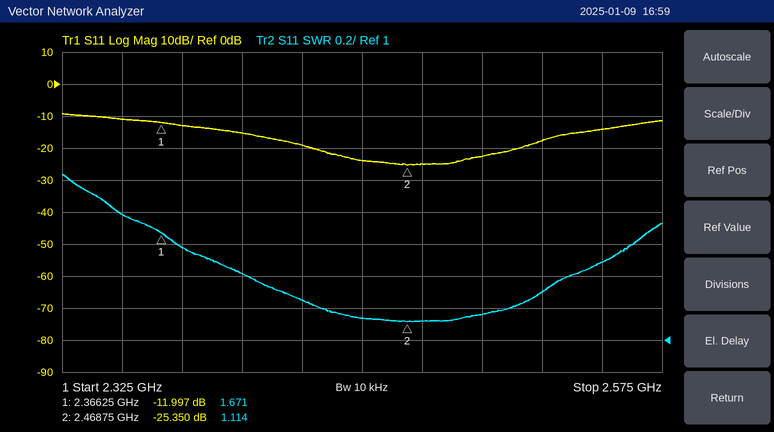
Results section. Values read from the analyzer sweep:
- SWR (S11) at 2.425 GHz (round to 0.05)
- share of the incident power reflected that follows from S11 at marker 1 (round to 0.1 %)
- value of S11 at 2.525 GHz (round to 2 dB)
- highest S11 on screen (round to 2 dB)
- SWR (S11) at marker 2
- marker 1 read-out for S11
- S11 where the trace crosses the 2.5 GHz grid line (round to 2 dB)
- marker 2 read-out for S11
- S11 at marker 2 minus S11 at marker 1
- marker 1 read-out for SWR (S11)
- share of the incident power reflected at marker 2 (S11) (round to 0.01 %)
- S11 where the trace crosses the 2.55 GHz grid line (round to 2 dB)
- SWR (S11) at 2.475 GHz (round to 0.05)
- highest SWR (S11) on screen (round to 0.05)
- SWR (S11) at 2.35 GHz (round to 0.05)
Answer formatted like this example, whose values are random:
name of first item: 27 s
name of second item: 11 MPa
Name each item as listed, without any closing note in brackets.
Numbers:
SWR (S11) at 2.425 GHz: 1.25
share of the incident power reflected that follows from S11 at marker 1: 6.3 %
value of S11 at 2.525 GHz: -18 dB
highest S11 on screen: -10 dB
SWR (S11) at marker 2: 1.114
marker 1 read-out for S11: -11.997 dB
S11 where the trace crosses the 2.5 GHz grid line: -22 dB
marker 2 read-out for S11: -25.350 dB
S11 at marker 2 minus S11 at marker 1: -13.353 dB
marker 1 read-out for SWR: 1.671
share of the incident power reflected at marker 2 (S11): 0.29 %
S11 where the trace crosses the 2.55 GHz grid line: -14 dB
SWR (S11) at 2.475 GHz: 1.10
highest SWR (S11) on screen: 2.05
SWR (S11) at 2.35 GHz: 1.80
